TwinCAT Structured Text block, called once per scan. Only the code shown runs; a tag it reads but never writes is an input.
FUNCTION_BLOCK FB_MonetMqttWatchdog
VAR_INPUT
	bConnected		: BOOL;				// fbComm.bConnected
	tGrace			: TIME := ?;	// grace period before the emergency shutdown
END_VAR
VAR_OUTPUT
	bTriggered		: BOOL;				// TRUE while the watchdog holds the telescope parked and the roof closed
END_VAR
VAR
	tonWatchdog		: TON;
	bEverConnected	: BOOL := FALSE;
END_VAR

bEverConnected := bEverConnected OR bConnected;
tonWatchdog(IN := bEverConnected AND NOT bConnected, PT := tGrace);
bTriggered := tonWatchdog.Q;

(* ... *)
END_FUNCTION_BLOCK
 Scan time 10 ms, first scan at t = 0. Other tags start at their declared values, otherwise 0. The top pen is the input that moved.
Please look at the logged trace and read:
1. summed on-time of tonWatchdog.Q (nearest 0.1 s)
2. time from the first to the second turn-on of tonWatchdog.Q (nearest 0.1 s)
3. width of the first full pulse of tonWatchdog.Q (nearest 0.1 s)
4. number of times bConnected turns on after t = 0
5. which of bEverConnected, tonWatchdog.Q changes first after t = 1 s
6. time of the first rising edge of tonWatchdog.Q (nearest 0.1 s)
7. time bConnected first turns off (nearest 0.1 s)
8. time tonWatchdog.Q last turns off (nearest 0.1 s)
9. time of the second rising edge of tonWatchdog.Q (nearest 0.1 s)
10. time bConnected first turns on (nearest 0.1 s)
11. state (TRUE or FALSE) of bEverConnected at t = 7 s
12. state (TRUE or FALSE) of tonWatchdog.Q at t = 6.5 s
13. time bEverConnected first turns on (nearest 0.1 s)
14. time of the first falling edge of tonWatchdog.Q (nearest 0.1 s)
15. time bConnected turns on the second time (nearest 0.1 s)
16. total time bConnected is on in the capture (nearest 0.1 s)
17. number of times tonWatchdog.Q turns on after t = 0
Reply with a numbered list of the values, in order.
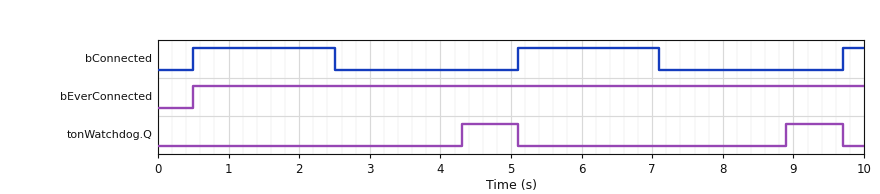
1. 1.6 s
2. 4.6 s
3. 0.8 s
4. 3
5. tonWatchdog.Q
6. 4.3 s
7. 2.5 s
8. 9.7 s
9. 8.9 s
10. 0.5 s
11. TRUE
12. FALSE
13. 0.5 s
14. 5.1 s
15. 5.1 s
16. 4.3 s
17. 2
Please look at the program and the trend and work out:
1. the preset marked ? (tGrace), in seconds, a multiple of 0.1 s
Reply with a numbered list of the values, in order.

1. 1.8 s
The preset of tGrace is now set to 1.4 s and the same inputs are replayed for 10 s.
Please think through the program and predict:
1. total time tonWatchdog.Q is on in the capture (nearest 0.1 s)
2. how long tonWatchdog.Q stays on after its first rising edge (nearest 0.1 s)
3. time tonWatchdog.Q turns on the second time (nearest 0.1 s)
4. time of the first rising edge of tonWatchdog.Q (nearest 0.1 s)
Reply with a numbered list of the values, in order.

1. 2.4 s
2. 1.2 s
3. 8.5 s
4. 3.9 s
